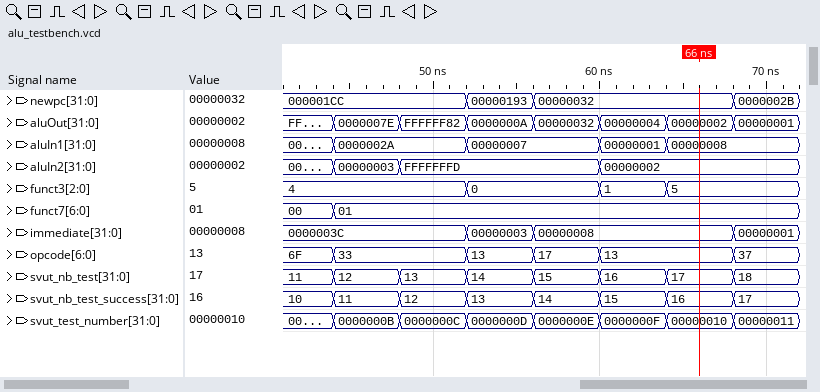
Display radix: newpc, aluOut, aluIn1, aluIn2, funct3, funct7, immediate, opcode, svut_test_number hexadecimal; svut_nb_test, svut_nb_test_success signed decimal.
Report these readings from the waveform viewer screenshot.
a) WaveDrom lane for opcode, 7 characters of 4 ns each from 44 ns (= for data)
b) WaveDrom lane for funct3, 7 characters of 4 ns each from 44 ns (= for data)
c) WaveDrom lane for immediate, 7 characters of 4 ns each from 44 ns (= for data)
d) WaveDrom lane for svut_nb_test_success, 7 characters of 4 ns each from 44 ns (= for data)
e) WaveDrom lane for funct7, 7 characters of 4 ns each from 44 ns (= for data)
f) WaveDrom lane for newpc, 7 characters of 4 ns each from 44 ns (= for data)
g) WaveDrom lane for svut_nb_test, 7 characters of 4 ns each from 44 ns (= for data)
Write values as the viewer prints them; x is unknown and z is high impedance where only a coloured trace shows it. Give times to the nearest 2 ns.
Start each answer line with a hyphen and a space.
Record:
- {name: 'opcode', wave: '=.===.=', data: '33 13 17 13 37'}
- {name: 'funct3', wave: '=.=.==.', data: '4 0 1 5'}
- {name: 'immediate', wave: '=.==..=', data: '0000003C 00000003 00000008 00000001'}
- {name: 'svut_nb_test_success', wave: '=======', data: '11 12 13 14 15 16 17'}
- {name: 'funct7', wave: '=......', data: '01'}
- {name: 'newpc', wave: '=.==..=', data: '000001CC 00000193 00000032 0000002B'}
- {name: 'svut_nb_test', wave: '=======', data: '12 13 14 15 16 17 18'}
